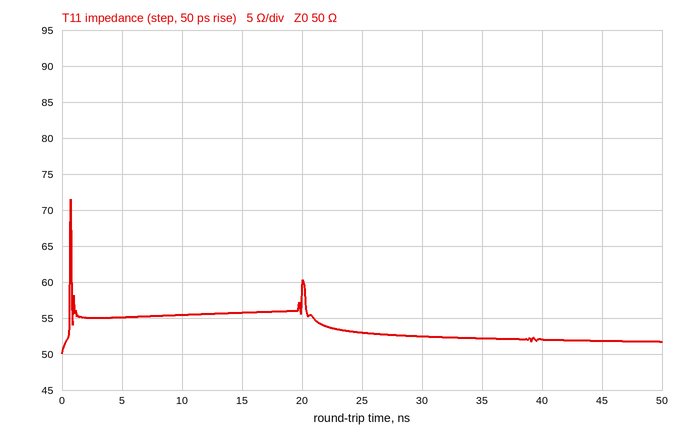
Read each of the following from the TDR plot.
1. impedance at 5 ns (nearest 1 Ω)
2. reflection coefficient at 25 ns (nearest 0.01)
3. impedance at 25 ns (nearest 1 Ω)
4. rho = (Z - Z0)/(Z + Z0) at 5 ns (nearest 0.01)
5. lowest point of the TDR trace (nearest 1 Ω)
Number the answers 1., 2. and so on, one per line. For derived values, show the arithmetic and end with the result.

1. 55 Ω
2. (53 − 50)/(53 + 50) ≈ +0.03
3. 53 Ω
4. (55 − 50)/(55 + 50) ≈ +0.05
5. 50 Ω
